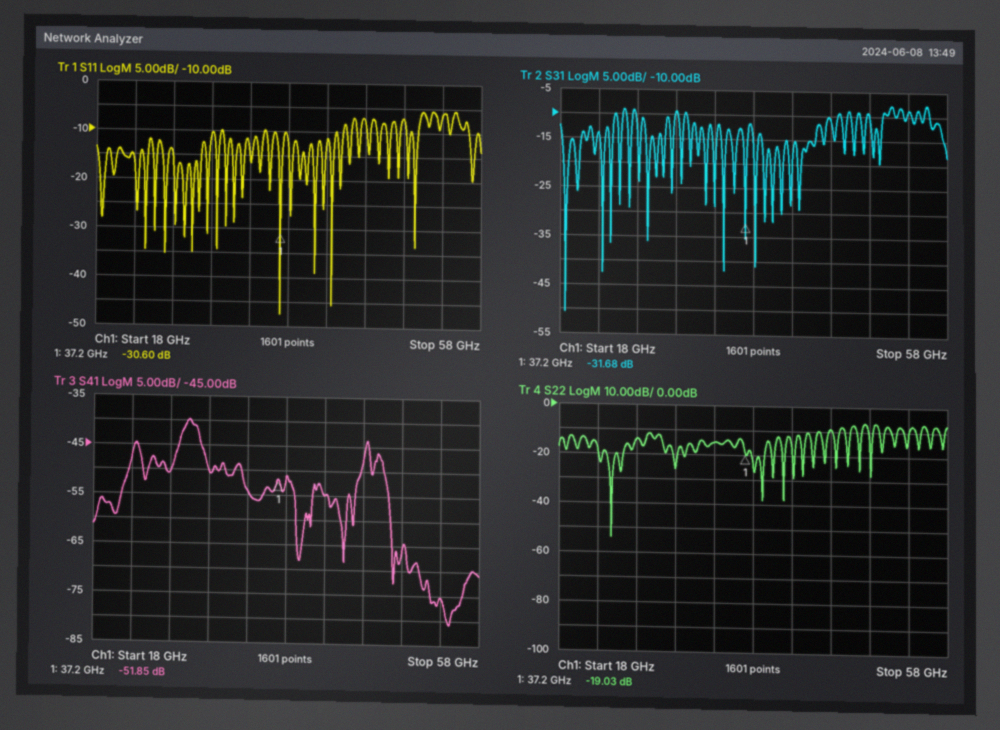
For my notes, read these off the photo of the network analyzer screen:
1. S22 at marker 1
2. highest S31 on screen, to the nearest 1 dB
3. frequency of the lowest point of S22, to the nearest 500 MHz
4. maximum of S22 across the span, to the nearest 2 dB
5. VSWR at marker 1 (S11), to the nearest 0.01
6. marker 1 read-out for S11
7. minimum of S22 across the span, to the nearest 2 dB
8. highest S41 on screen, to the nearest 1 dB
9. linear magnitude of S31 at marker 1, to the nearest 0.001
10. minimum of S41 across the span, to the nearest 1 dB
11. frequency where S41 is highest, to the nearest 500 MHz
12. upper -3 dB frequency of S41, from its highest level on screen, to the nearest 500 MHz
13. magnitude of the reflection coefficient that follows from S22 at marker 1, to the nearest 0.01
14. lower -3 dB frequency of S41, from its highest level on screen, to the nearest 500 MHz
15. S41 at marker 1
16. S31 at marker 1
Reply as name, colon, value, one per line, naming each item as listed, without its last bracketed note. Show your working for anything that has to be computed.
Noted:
S22 at marker 1: -19.03 dB
highest S31 on screen, to the nearest 1 dB: -8 dB
frequency of the lowest point of S22, to the nearest 500 MHz: 23.5 GHz
maximum of S22 across the span, to the nearest 2 dB: -6 dB
VSWR at marker 1 (S11), to the nearest 0.01: (1 + 0.0295)/(1 − 0.0295) ≈ 1.06
marker 1 read-out for S11: -30.60 dB
minimum of S22 across the span, to the nearest 2 dB: -54 dB
highest S41 on screen, to the nearest 1 dB: -40 dB
linear magnitude of S31 at marker 1, to the nearest 0.001: 10^(-31.68/20) ≈ 0.026
minimum of S41 across the span, to the nearest 1 dB: -81 dB
frequency where S41 is highest, to the nearest 500 MHz: 28.0 GHz
upper -3 dB frequency of S41, from its highest level on screen, to the nearest 500 MHz: 29.0 GHz
magnitude of the reflection coefficient that follows from S22 at marker 1, to the nearest 0.01: 10^(-19.03/20) ≈ 0.11
lower -3 dB frequency of S41, from its highest level on screen, to the nearest 500 MHz: 27.0 GHz
S41 at marker 1: -51.85 dB
S31 at marker 1: -31.68 dB
